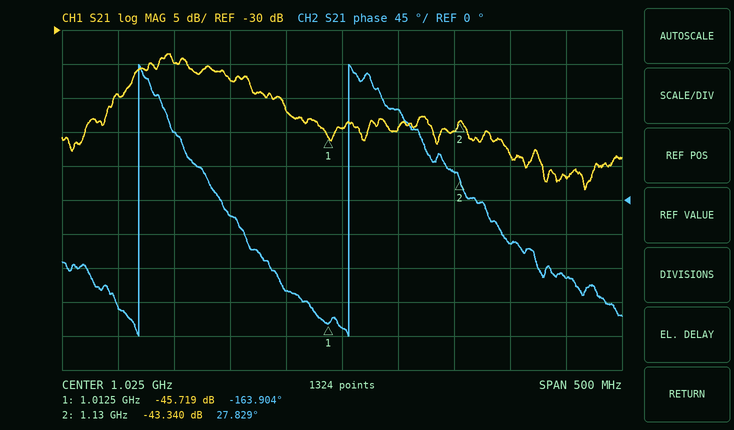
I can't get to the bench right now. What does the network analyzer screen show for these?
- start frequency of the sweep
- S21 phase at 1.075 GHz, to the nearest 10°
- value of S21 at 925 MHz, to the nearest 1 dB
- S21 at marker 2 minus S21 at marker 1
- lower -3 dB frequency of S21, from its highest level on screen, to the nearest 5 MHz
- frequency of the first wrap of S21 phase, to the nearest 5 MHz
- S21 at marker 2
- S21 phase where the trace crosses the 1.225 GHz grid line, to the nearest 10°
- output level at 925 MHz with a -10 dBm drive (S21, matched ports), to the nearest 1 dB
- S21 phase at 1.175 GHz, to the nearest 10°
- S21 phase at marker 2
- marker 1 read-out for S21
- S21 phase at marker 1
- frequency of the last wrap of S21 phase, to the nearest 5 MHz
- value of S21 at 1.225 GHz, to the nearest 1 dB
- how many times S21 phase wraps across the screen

775 MHz
120°
-37 dB
2.379 dB
840 MHz
845 MHz
-43.340 dB
-100°
-47 dBm
-60°
27.829°
-45.719 dB
-163.904°
1.030 GHz
-52 dB
2
